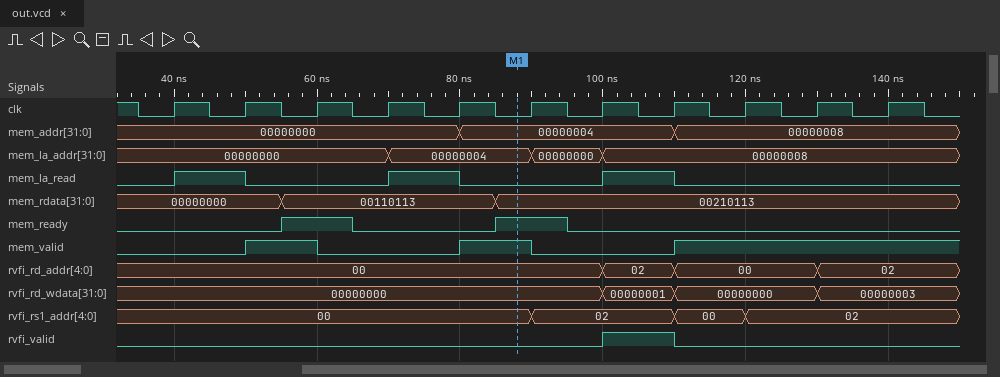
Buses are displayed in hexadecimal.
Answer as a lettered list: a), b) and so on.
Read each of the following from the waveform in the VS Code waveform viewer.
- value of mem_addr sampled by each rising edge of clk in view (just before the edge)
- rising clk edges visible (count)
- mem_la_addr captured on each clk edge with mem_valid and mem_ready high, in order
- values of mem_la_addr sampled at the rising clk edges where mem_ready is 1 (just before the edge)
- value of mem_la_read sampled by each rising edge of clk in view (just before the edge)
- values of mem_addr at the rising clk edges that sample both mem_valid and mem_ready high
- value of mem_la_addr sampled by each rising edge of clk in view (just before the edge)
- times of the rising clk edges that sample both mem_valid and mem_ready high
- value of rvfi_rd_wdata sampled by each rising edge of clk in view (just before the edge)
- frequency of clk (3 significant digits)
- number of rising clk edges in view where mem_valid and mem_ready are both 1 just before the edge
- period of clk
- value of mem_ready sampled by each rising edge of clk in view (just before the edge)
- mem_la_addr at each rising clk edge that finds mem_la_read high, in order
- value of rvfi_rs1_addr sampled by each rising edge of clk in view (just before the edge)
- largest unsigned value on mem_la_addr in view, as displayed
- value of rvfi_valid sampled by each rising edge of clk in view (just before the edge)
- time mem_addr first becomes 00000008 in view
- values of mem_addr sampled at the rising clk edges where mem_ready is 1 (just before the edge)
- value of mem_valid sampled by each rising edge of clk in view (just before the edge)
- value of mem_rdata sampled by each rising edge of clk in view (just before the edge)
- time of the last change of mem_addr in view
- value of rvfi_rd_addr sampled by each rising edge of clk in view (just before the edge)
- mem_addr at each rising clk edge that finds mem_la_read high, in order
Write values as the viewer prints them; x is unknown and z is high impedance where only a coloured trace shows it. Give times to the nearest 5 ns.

a) 00000000, 00000000, 00000000, 00000000, 00000000, 00000004, 00000004, 00000004, 00000008, 00000008, 00000008
b) 11
c) 00000000, 00000004
d) 00000000, 00000004
e) 0 1 0 0 1 0 0 1 0 0 0
f) 00000000, 00000004
g) 00000000, 00000000, 00000000, 00000000, 00000004, 00000004, 00000000, 00000008, 00000008, 00000008, 00000008
h) 60 ns, 90 ns
i) 00000000, 00000000, 00000000, 00000000, 00000000, 00000000, 00000000, 00000001, 00000000, 00000000, 00000003
j) 100 MHz
k) 2
l) 10 ns
m) 0 0 1 0 0 1 0 0 0 0 0
n) 00000000, 00000004, 00000008
o) 00, 00, 00, 00, 00, 00, 02, 02, 00, 02, 02
p) 00000008
q) 0 0 0 0 0 0 0 1 0 0 0
r) 110 ns
s) 00000000, 00000004
t) 0 0 1 0 0 1 0 0 1 1 1
u) 00000000, 00000000, 00110113, 00110113, 00110113, 00210113, 00210113, 00210113, 00210113, 00210113, 00210113
v) 110 ns
w) 00, 00, 00, 00, 00, 00, 00, 02, 00, 00, 02
x) 00000000, 00000000, 00000004
